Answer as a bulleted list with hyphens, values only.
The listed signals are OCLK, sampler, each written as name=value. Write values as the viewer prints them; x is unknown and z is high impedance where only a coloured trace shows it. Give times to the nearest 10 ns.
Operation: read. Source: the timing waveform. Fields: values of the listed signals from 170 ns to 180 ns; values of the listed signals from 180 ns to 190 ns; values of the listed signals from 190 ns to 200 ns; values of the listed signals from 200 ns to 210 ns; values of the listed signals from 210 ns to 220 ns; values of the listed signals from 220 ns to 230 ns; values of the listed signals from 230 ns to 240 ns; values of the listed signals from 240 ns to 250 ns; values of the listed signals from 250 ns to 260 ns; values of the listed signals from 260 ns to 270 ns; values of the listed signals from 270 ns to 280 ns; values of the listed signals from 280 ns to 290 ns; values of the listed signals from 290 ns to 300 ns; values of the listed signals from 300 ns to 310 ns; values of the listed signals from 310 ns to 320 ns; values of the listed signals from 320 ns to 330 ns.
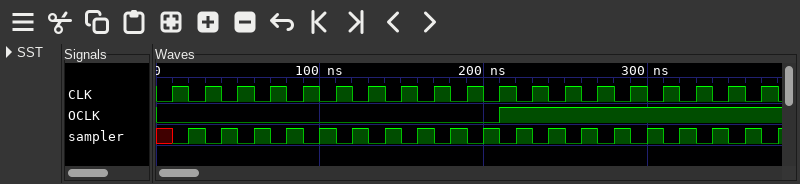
- OCLK=0, sampler=0
- OCLK=0, sampler=1
- OCLK=0, sampler=0
- OCLK=0, sampler=1
- OCLK=1, sampler=0
- OCLK=1, sampler=1
- OCLK=1, sampler=0
- OCLK=1, sampler=1
- OCLK=1, sampler=0
- OCLK=1, sampler=1
- OCLK=1, sampler=0
- OCLK=1, sampler=1
- OCLK=1, sampler=0
- OCLK=1, sampler=1
- OCLK=1, sampler=0
- OCLK=1, sampler=1
